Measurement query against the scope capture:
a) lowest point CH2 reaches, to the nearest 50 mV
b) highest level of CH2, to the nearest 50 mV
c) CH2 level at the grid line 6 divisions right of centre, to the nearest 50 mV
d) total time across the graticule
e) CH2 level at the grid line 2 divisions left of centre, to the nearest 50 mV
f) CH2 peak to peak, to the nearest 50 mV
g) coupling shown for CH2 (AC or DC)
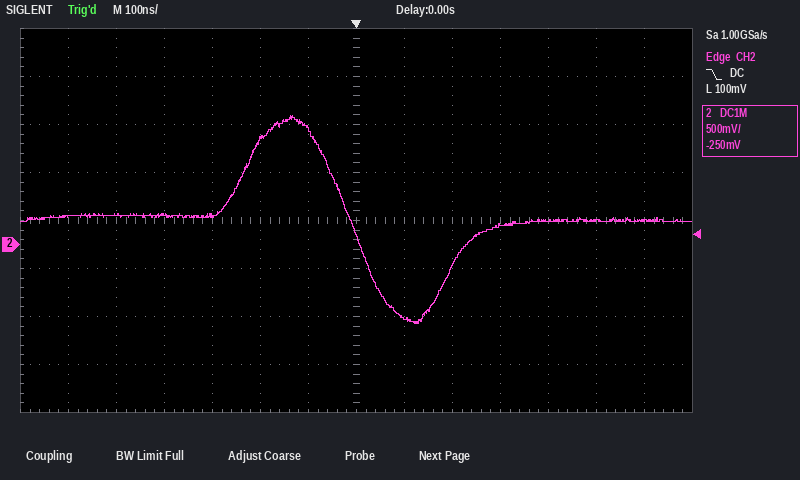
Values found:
-800 mV
1.35 V
250 mV
1.4 µs
1.10 V
2.15 V
DC
